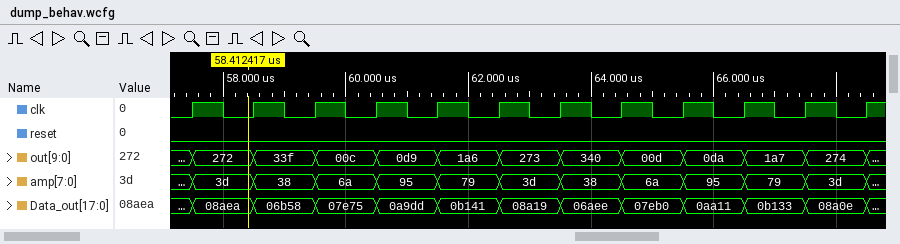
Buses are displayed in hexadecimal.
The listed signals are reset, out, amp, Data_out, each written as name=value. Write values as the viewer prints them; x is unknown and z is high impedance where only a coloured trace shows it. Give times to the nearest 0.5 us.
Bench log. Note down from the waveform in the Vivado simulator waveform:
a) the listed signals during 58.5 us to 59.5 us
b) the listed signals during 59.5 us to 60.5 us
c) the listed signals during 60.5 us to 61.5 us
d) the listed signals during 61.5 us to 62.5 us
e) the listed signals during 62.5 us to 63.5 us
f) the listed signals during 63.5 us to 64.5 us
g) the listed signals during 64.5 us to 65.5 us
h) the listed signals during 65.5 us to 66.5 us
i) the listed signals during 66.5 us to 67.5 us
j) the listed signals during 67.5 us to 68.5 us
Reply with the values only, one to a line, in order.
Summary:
reset=0, out=33f, amp=38, Data_out=06b58
reset=0, out=00c, amp=6a, Data_out=07e75
reset=0, out=0d9, amp=95, Data_out=0a9dd
reset=0, out=1a6, amp=79, Data_out=0b141
reset=0, out=273, amp=3d, Data_out=08a19
reset=0, out=340, amp=38, Data_out=06aee
reset=0, out=00d, amp=6a, Data_out=07eb0
reset=0, out=0da, amp=95, Data_out=0aa11
reset=0, out=1a7, amp=79, Data_out=0b133
reset=0, out=274, amp=3d, Data_out=08a0e
